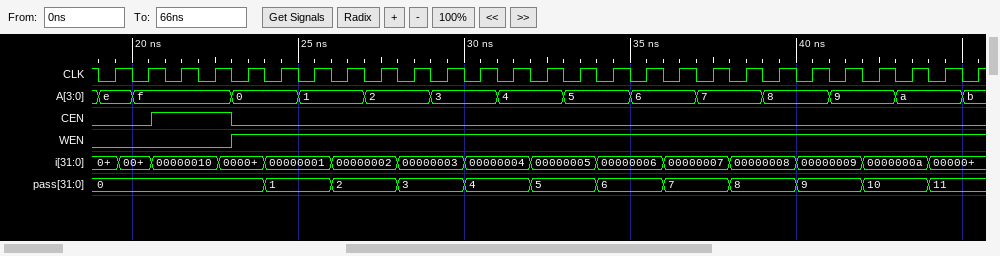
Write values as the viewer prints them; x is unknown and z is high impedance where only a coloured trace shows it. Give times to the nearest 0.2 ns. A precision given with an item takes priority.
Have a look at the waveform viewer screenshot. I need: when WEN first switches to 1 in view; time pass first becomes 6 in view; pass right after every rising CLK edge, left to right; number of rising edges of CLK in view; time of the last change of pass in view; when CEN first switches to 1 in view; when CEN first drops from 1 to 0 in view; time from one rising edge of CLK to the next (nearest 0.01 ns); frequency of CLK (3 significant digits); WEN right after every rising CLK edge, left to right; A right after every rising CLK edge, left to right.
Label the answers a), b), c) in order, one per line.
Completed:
a) 23 ns
b) 34 ns
c) 0, 0, 0, 0, 0, 1, 1, 2, 2, 3, 3, 4, 4, 5, 5, 6, 6, 7, 7, 8, 8, 9, 9, 10, 10, 11, 11
d) 27
e) 44 ns
f) 20.6 ns
g) 23 ns
h) 1 ns
i) 1.00 GHz
j) 0 0 0 0 1 1 1 1 1 1 1 1 1 1 1 1 1 1 1 1 1 1 1 1 1 1 1
k) e, f, f, f, 0, 0, 1, 1, 2, 2, 3, 3, 4, 4, 5, 5, 6, 6, 7, 7, 8, 8, 9, 9, a, a, b
